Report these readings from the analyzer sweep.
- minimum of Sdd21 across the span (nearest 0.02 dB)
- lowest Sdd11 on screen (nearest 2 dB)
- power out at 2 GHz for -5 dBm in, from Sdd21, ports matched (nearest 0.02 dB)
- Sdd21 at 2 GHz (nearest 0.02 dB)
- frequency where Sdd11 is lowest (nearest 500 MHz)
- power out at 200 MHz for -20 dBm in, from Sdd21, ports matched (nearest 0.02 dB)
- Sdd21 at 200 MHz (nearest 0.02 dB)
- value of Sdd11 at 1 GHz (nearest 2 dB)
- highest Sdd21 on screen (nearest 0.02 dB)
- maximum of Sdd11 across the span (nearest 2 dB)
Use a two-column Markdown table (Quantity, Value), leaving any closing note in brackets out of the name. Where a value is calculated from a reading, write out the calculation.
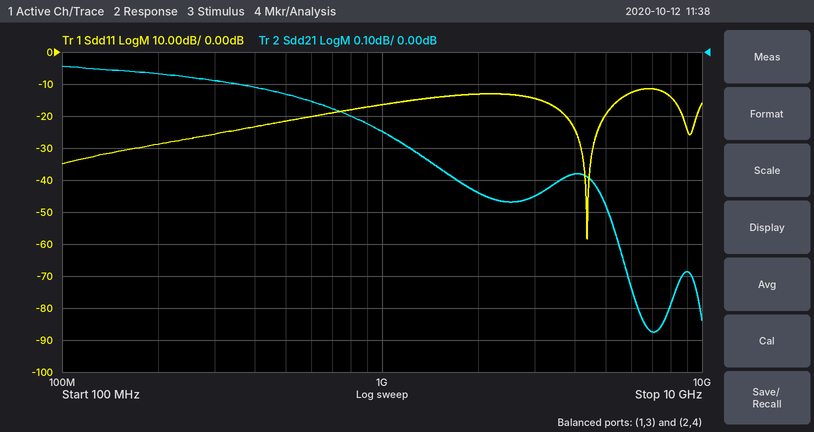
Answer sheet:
| Quantity | Value |
|---|---|
| minimum of Sdd21 across the span | -0.88 dB |
| lowest Sdd11 on screen | -58 dB |
| power out at 2 GHz for -5 dBm in, from Sdd21, ports matched | -5 dBm + (-0.44 dB) = -5.44 dBm |
| Sdd21 at 2 GHz | -0.44 dB |
| frequency where Sdd11 is lowest | 4.5 GHz |
| power out at 200 MHz for -20 dBm in, from Sdd21, ports matched | -20 dBm + (-0.06 dB) = -20.06 dBm |
| Sdd21 at 200 MHz | -0.06 dB |
| value of Sdd11 at 1 GHz | -16 dB |
| highest Sdd21 on screen | -0.04 dB |
| maximum of Sdd11 across the span | -12 dB |
